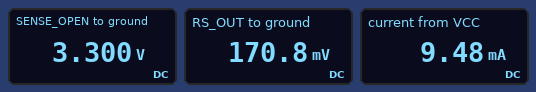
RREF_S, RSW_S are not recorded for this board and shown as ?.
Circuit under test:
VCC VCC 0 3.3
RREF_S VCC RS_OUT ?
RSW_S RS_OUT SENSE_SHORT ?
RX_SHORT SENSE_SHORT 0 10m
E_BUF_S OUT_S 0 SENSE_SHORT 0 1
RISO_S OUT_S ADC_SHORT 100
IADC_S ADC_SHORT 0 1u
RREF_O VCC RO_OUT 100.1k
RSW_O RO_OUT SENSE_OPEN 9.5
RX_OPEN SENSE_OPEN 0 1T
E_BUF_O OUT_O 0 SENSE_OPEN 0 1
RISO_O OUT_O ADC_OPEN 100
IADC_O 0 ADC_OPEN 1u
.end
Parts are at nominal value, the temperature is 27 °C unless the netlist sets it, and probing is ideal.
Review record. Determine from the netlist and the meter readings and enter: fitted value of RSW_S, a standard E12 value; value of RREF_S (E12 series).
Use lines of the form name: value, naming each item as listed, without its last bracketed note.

fitted value of RSW_S, a standard E12 value: 18 Ω
value of RREF_S: 330 Ω
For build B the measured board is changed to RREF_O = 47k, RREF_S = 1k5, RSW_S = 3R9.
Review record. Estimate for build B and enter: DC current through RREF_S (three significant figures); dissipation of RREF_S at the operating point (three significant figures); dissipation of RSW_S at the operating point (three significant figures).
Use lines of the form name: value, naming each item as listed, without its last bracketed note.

DC current through RREF_S: 2.19 mA
dissipation of RREF_S at the operating point: 7.22 mW
dissipation of RSW_S at the operating point: 18.8 µW
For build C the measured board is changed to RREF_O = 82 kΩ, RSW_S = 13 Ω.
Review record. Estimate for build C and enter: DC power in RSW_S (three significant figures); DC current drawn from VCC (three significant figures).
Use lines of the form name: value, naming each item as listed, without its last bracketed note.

DC power in RSW_S: 1.20 mW
DC current drawn from VCC: 9.62 mA
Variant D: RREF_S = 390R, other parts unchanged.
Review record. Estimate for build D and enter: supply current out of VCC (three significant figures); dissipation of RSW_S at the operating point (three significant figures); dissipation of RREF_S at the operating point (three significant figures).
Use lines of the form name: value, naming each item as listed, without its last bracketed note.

supply current out of VCC: 8.09 mA
dissipation of RSW_S at the operating point: 1.18 mW
dissipation of RREF_S at the operating point: 25.5 mW
